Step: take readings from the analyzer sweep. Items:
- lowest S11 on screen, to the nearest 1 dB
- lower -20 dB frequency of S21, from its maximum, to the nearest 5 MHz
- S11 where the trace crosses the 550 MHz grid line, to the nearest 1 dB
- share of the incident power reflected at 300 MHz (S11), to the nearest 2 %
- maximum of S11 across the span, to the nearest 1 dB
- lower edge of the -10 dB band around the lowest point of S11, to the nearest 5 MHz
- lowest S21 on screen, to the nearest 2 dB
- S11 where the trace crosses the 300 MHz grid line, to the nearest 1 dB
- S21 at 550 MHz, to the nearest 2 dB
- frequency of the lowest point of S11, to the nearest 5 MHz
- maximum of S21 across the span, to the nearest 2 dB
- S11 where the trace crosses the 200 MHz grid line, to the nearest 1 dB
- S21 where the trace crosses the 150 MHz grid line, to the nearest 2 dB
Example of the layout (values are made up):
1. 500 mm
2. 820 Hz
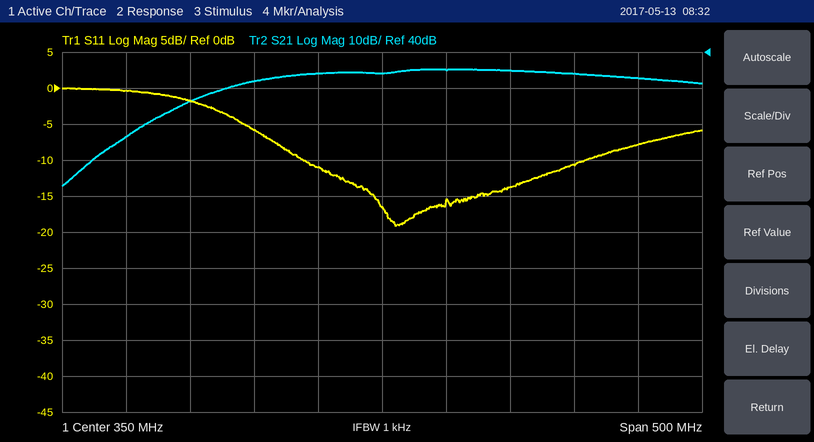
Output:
1. -19 dB
2. 145 MHz
3. -8 dB
4. 8 %
5. 0 dB
6. 290 MHz
7. 2 dB
8. -11 dB
9. 32 dB
10. 360 MHz
11. 36 dB
12. -2 dB
13. 16 dB
